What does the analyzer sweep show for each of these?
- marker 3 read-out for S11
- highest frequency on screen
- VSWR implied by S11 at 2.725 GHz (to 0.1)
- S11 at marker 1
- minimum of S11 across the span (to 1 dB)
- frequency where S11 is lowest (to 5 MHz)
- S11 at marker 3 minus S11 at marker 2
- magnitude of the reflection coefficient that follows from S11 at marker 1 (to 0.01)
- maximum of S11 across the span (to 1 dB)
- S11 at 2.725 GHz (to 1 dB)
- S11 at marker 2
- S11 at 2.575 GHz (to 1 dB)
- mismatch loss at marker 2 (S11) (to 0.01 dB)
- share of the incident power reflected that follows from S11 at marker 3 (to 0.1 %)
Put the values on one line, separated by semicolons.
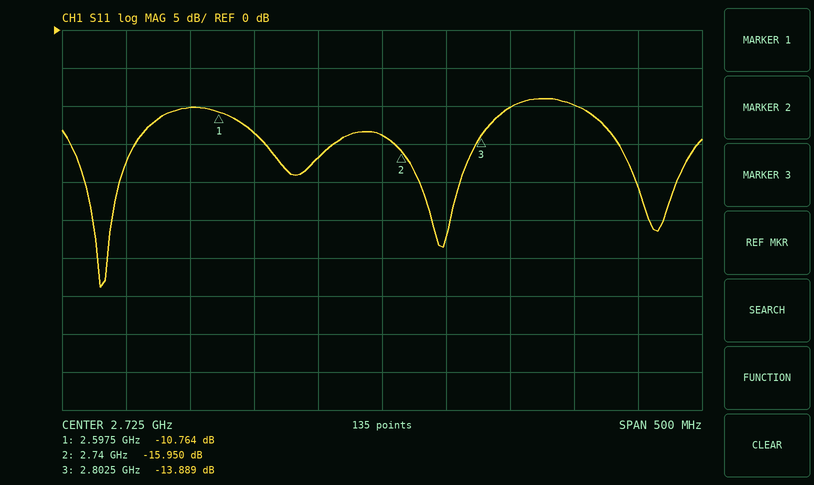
-13.889 dB; 2.975 GHz; 1.5; -10.764 dB; -34 dB; 2.505 GHz; 2.061 dB; 0.29; -9 dB; -14 dB; -15.950 dB; -10 dB; 0.11 dB; 4.1 %
